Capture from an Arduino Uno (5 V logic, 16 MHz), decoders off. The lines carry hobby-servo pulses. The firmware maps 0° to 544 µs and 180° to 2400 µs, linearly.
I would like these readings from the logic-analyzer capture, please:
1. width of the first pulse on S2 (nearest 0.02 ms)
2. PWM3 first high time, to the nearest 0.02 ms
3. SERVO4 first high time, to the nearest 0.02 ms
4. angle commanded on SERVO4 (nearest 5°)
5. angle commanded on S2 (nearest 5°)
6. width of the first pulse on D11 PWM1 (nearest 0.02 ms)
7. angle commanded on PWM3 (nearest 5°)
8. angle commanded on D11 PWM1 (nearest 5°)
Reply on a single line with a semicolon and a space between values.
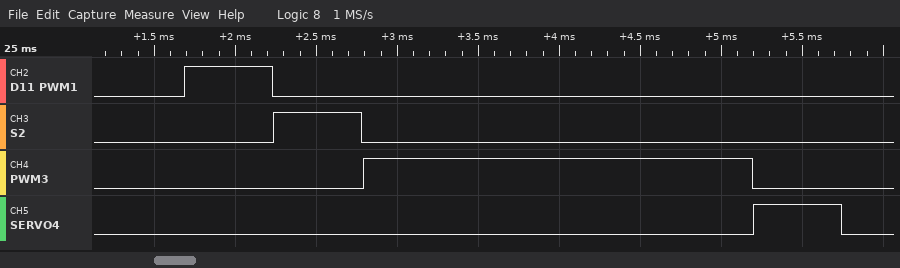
0.54 ms; 2.40 ms; 0.54 ms; 0°; 0°; 0.54 ms; 180°; 0°
